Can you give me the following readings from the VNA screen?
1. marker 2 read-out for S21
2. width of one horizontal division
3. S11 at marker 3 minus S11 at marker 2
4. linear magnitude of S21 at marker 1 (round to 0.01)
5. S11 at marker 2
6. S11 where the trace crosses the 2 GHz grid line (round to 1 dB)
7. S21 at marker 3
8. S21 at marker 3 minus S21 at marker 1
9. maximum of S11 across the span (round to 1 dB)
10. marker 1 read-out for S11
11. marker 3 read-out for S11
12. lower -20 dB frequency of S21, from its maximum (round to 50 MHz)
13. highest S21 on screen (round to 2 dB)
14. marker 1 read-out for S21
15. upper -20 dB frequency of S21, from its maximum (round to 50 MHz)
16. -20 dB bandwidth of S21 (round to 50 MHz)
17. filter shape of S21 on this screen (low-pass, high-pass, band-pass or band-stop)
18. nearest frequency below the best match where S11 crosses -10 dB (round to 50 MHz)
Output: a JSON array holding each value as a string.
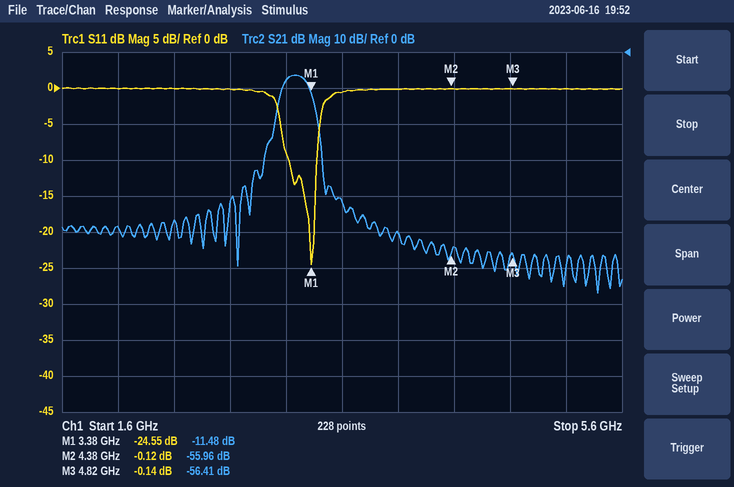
["-55.96 dB", "400 MHz", "-0.02 dB", "0.27", "-0.12 dB", "0 dB", "-56.41 dB", "-44.93 dB", "0 dB", "-24.55 dB", "-0.14 dB", "3.05 GHz", "-6 dB", "-11.48 dB", "3.45 GHz", "400 MHz", "band-pass", "3.20 GHz"]
